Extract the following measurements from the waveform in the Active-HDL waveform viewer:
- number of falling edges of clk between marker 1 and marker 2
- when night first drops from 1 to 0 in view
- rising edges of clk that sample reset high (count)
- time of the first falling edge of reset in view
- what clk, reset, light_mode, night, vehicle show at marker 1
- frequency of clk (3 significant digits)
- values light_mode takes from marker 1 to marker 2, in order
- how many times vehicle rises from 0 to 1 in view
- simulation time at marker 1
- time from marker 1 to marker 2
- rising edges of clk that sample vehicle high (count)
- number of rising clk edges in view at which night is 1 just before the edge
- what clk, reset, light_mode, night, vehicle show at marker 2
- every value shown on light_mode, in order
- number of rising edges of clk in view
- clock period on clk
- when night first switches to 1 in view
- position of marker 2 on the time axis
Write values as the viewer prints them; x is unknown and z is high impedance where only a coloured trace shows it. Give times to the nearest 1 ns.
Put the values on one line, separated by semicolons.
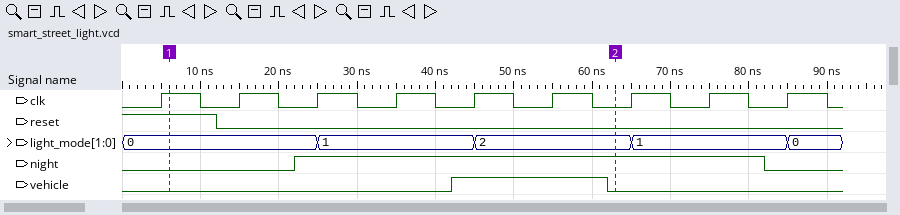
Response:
6; 82 ns; 1; 12 ns; clk=1, reset=1, light_mode=0, night=0, vehicle=0; 100 MHz; 0, 1, 2; 1; 6 ns; 57 ns; 2; 6; clk=0, reset=0, light_mode=2, night=1, vehicle=0; 0, 1, 2, 1, 0; 9; 10 ns; 22 ns; 63 ns
